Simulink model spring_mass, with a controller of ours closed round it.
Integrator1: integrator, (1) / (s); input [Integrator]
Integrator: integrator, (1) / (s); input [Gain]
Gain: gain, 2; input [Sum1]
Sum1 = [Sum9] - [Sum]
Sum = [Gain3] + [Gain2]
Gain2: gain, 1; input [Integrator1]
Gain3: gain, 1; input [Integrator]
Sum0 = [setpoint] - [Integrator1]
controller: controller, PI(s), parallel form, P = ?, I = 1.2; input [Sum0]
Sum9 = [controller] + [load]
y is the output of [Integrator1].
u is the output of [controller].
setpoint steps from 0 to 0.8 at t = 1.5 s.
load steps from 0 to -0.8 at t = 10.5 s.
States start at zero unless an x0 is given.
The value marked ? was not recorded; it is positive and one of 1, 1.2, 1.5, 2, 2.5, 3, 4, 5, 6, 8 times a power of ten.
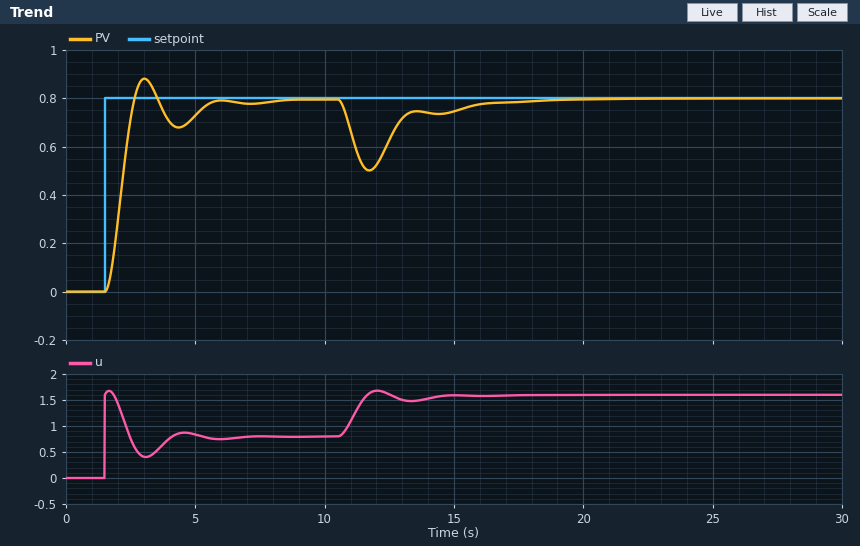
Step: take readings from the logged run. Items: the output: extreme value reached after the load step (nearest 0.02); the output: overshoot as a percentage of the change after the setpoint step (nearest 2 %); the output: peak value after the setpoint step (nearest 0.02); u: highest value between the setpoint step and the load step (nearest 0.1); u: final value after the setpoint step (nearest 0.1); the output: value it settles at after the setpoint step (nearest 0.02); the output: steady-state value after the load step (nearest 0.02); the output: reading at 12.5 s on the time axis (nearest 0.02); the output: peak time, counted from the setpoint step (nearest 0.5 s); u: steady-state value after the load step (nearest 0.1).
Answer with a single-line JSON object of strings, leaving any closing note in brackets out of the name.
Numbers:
{"the output: extreme value reached after the load step": "0.50", "the output: overshoot as a percentage of the change after the setpoint step": "10 %", "the output: peak value after the setpoint step": "0.88", "u: highest value between the setpoint step and the load step": "1.7", "u: final value after the setpoint step": "0.8", "the output: value it settles at after the setpoint step": "0.80", "the output: steady-state value after the load step": "0.80", "the output: reading at 12.5 s on the time axis": "0.62", "the output: peak time, counted from the setpoint step": "1.5 s", "u: steady-state value after the load step": "1.6"}
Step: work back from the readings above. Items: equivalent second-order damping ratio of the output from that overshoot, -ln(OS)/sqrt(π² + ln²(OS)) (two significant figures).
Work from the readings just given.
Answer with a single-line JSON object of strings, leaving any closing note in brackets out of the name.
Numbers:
{"equivalent second-order damping ratio of the output from that overshoot, -ln(OS)/sqrt(π² + ln²(OS))": "0.59"}
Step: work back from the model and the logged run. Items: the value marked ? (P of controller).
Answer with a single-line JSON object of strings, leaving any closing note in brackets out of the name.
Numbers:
{"the value marked ?": "2"}
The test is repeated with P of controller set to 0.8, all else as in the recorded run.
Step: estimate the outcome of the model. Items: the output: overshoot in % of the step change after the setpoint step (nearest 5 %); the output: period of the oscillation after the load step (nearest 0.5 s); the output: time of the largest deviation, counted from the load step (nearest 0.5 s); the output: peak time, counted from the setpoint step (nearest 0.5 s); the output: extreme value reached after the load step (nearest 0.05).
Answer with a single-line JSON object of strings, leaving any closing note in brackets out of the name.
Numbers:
{"the output: overshoot in % of the step change after the setpoint step": "15 %", "the output: period of the oscillation after the load step": "4.5 s", "the output: time of the largest deviation, counted from the load step": "1.5 s", "the output: peak time, counted from the setpoint step": "2.5 s", "the output: extreme value reached after the load step": "0.40"}
